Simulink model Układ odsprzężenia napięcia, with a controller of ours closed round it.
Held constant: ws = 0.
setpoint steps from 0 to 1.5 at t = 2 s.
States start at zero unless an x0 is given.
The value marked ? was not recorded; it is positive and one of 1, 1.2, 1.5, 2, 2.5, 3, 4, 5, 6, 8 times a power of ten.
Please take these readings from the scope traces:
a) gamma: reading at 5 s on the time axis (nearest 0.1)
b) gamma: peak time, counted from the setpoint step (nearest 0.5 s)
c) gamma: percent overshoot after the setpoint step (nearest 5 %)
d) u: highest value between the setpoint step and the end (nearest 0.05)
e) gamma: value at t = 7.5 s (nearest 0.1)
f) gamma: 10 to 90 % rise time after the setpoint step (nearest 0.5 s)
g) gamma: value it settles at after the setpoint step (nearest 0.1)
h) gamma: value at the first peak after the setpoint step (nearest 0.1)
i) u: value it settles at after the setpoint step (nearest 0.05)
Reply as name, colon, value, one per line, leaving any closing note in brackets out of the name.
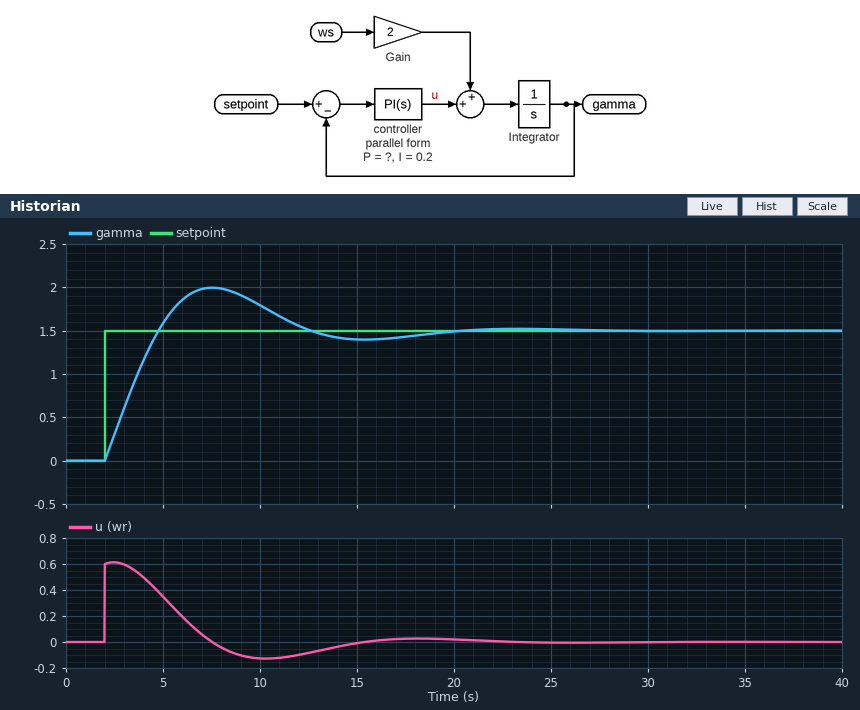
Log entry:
gamma: reading at 5 s on the time axis: 1.6
gamma: peak time, counted from the setpoint step: 5.5 s
gamma: percent overshoot after the setpoint step: 35 %
u: highest value between the setpoint step and the end: 0.60
gamma: value at t = 7.5 s: 2.0
gamma: 10 to 90 % rise time after the setpoint step: 2.0 s
gamma: value it settles at after the setpoint step: 1.5
gamma: value at the first peak after the setpoint step: 2.0
u: value it settles at after the setpoint step: 0.00
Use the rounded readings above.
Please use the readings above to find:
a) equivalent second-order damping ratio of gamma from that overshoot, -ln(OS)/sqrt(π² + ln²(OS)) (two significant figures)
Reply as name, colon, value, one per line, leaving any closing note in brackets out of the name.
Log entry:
equivalent second-order damping ratio of gamma from that overshoot, -ln(OS)/sqrt(π² + ln²(OS)): 0.32
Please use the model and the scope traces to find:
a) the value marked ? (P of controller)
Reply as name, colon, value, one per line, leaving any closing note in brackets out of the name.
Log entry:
the value marked ?: 0.4
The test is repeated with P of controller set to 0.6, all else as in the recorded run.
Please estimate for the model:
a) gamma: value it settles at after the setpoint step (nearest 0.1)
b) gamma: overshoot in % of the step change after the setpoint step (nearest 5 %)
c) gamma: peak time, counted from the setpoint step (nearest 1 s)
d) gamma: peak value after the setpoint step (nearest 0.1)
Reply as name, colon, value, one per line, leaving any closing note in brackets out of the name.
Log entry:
gamma: value it settles at after the setpoint step: 1.5
gamma: overshoot in % of the step change after the setpoint step: 20 %
gamma: peak time, counted from the setpoint step: 5 s
gamma: peak value after the setpoint step: 1.8
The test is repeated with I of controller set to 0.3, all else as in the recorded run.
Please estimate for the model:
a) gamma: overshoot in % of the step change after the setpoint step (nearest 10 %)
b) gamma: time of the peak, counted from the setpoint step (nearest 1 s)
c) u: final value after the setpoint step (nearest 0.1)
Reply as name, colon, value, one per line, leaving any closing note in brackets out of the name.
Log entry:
gamma: overshoot in % of the step change after the setpoint step: 40 %
gamma: time of the peak, counted from the setpoint step: 5 s
u: final value after the setpoint step: 0.0
